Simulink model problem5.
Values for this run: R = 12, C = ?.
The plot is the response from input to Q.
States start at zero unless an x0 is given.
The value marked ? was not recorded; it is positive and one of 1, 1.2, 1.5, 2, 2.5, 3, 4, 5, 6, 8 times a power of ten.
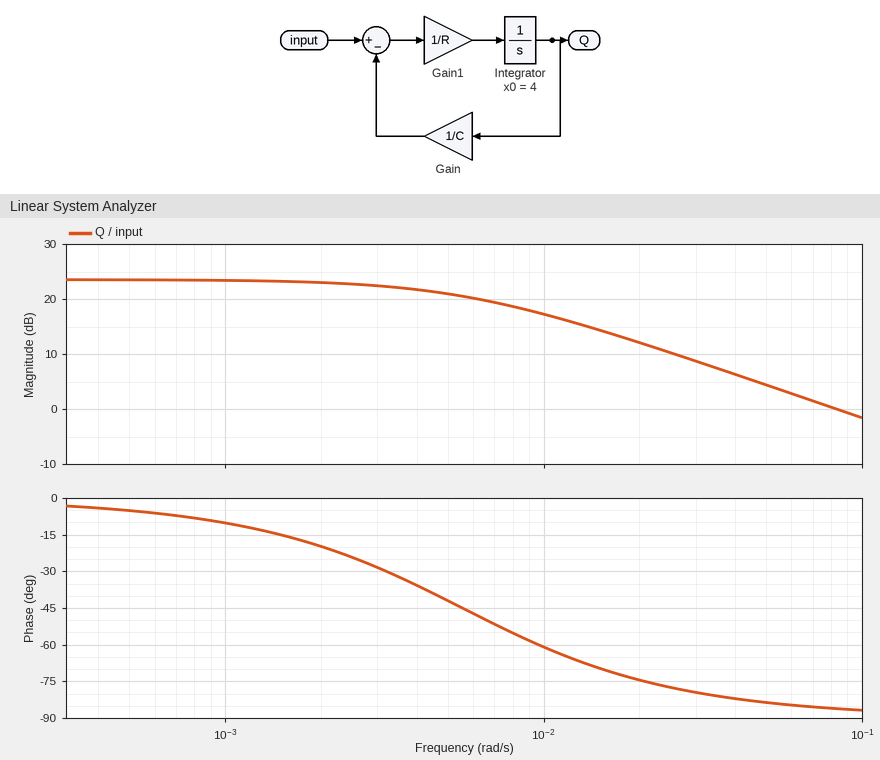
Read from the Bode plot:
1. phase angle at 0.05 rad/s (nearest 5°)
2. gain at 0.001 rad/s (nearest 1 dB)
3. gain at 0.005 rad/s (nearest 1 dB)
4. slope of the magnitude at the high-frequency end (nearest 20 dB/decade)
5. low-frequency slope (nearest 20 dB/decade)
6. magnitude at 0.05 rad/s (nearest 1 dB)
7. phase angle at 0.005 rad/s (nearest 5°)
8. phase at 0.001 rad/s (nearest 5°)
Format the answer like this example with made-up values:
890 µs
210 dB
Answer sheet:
-85°
23 dB
21 dB
-20 dB/decade
0 dB/decade
4 dB
-40°
-10°
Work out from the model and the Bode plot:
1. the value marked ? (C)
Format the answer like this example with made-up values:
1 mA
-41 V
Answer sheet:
15
